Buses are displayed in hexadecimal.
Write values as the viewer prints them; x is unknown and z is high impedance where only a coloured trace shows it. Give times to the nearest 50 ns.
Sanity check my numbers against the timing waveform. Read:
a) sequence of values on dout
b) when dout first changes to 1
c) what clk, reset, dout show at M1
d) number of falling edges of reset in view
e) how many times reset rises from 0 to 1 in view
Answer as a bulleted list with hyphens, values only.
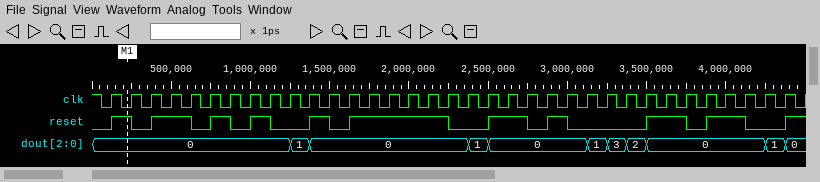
- 0, 1, 0, 1, 0, 1, 3, 2, 0, 1, 0
- 1250 ns
- clk=0, reset=1, dout=0
- 10
- 11
